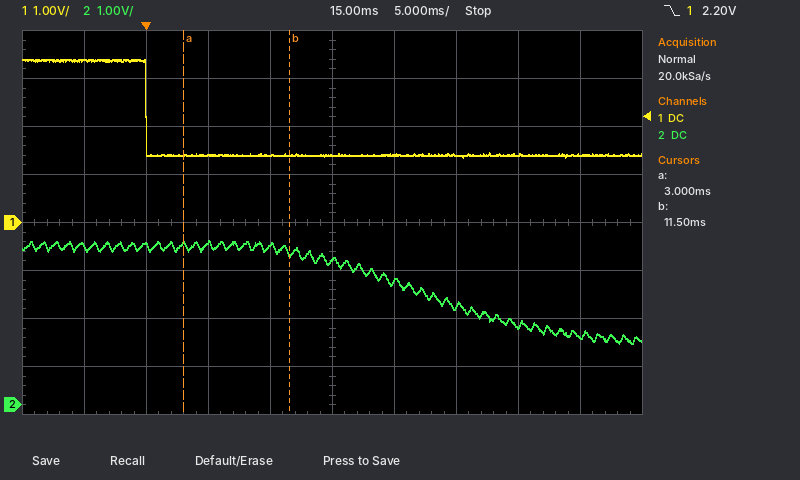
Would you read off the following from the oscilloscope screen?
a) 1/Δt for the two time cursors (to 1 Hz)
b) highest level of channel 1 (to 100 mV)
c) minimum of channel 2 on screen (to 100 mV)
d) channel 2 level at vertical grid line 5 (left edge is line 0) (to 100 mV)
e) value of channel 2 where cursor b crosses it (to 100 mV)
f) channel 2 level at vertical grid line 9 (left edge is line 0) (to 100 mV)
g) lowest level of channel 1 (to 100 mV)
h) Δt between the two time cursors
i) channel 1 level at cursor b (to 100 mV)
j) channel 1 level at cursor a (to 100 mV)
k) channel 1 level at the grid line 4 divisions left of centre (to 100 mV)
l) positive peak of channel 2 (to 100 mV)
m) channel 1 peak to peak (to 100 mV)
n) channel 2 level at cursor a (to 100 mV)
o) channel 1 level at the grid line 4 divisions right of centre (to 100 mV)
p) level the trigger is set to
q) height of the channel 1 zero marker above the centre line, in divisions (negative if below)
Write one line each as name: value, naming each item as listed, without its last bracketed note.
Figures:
1/Δt for the two time cursors: 118 Hz
highest level of channel 1: 3.4 V
minimum of channel 2 on screen: 1.3 V
channel 2 level at vertical grid line 5 (left edge is line 0): 3.0 V
value of channel 2 where cursor b crosses it: 3.2 V
channel 2 level at vertical grid line 9 (left edge is line 0): 1.4 V
lowest level of channel 1: 1.4 V
Δt between the two time cursors: 8.5 ms
channel 1 level at cursor b: 1.4 V
channel 1 level at cursor a: 1.4 V
channel 1 level at the grid line 4 divisions left of centre: 3.4 V
positive peak of channel 2: 3.4 V
channel 1 peak to peak: 2.0 V
channel 2 level at cursor a: 3.3 V
channel 1 level at the grid line 4 divisions right of centre: 1.4 V
level the trigger is set to: 2.20 V
height of the channel 1 zero marker above the centre line, in divisions: 0.0 div
